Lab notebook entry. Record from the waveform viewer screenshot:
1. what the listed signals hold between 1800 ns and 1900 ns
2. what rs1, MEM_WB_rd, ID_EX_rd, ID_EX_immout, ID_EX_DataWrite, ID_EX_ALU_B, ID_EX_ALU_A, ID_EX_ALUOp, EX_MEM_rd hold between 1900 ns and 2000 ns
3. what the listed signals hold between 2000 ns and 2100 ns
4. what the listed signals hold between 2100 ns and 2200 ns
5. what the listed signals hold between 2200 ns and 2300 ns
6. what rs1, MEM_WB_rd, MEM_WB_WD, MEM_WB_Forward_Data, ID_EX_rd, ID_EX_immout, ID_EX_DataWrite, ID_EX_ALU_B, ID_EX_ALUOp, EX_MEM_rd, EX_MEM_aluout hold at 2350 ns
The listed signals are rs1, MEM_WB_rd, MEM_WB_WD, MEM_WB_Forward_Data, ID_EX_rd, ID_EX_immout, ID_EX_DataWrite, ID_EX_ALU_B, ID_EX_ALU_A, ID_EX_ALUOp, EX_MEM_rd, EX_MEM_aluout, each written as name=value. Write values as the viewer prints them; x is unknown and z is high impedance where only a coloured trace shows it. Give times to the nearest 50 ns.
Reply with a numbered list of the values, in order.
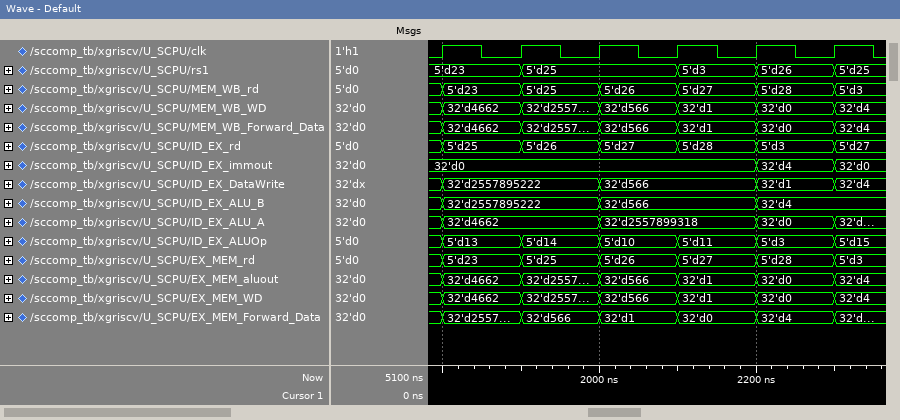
1. rs1=5'd23, MEM_WB_rd=5'd23, MEM_WB_WD=32'd4662, MEM_WB_Forward_Data=32'd4662, ID_EX_rd=5'd25, ID_EX_immout=32'd0, ID_EX_DataWrite=32'd2557895222, ID_EX_ALU_B=32'd2557895222, ID_EX_ALU_A=32'd4662, ID_EX_ALUOp=5'd13, EX_MEM_rd=5'd23, EX_MEM_aluout=32'd4662
2. rs1=5'd25, MEM_WB_rd=5'd25, ID_EX_rd=5'd26, ID_EX_immout=32'd0, ID_EX_DataWrite=32'd2557895222, ID_EX_ALU_B=32'd2557895222, ID_EX_ALU_A=32'd4662, ID_EX_ALUOp=5'd14, EX_MEM_rd=5'd25
3. rs1=5'd25, MEM_WB_rd=5'd26, MEM_WB_WD=32'd566, MEM_WB_Forward_Data=32'd566, ID_EX_rd=5'd27, ID_EX_immout=32'd0, ID_EX_DataWrite=32'd566, ID_EX_ALU_B=32'd566, ID_EX_ALU_A=32'd2557899318, ID_EX_ALUOp=5'd10, EX_MEM_rd=5'd26, EX_MEM_aluout=32'd566
4. rs1=5'd3, MEM_WB_rd=5'd27, MEM_WB_WD=32'd1, MEM_WB_Forward_Data=32'd1, ID_EX_rd=5'd28, ID_EX_immout=32'd0, ID_EX_DataWrite=32'd566, ID_EX_ALU_B=32'd566, ID_EX_ALU_A=32'd2557899318, ID_EX_ALUOp=5'd11, EX_MEM_rd=5'd27, EX_MEM_aluout=32'd1
5. rs1=5'd26, MEM_WB_rd=5'd28, MEM_WB_WD=32'd0, MEM_WB_Forward_Data=32'd0, ID_EX_rd=5'd3, ID_EX_immout=32'd4, ID_EX_DataWrite=32'd1, ID_EX_ALU_B=32'd4, ID_EX_ALU_A=32'd0, ID_EX_ALUOp=5'd3, EX_MEM_rd=5'd28, EX_MEM_aluout=32'd0
6. rs1=5'd25, MEM_WB_rd=5'd3, MEM_WB_WD=32'd4, MEM_WB_Forward_Data=32'd4, ID_EX_rd=5'd27, ID_EX_immout=32'd0, ID_EX_DataWrite=32'd4, ID_EX_ALU_B=32'd4, ID_EX_ALUOp=5'd15, EX_MEM_rd=5'd3, EX_MEM_aluout=32'd4
